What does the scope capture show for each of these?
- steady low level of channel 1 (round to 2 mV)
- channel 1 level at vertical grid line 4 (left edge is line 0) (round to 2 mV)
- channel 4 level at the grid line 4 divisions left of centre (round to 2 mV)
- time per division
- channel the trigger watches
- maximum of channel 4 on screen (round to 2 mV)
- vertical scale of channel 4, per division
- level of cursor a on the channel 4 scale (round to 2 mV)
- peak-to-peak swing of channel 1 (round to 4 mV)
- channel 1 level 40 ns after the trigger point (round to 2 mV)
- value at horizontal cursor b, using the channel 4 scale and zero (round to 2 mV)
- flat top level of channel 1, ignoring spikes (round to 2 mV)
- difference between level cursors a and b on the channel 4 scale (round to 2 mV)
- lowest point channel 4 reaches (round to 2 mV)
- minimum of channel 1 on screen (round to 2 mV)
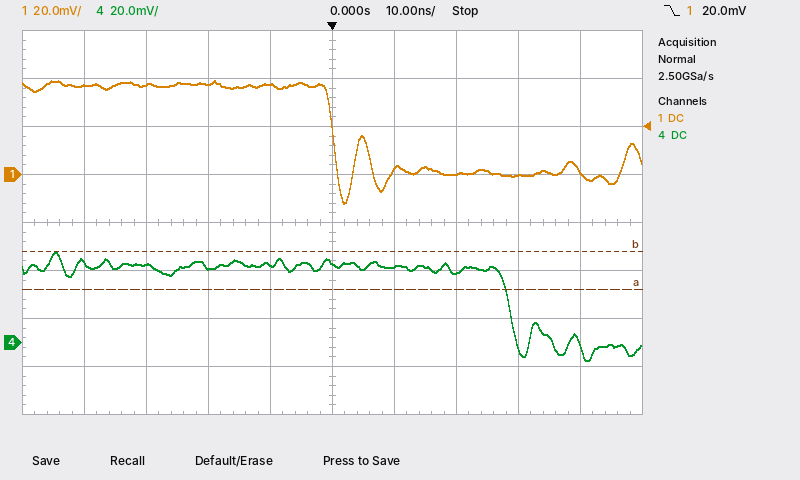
0 mV
38 mV
34 mV
10 ns
channel 1
38 mV
20 mV
22 mV
52 mV
2 mV
38 mV
38 mV
16 mV
-8 mV
-12 mV
